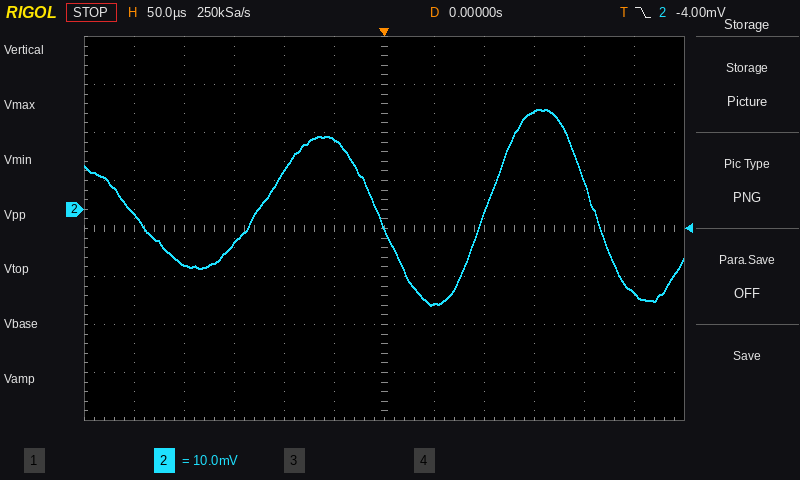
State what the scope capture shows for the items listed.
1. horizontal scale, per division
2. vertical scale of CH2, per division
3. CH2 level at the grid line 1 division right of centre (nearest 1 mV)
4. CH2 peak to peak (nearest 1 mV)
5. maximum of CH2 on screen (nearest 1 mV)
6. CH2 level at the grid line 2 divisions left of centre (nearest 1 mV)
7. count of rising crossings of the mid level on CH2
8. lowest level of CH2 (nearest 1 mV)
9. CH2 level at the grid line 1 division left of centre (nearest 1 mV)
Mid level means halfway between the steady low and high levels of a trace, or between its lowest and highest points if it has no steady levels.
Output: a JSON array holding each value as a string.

["50 µs", "10 mV", "-20 mV", "41 mV", "21 mV", "8 mV", "2", "-20 mV", "15 mV"]
